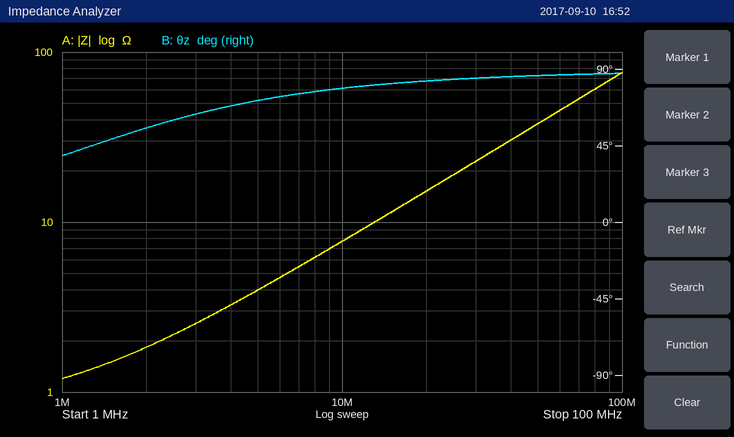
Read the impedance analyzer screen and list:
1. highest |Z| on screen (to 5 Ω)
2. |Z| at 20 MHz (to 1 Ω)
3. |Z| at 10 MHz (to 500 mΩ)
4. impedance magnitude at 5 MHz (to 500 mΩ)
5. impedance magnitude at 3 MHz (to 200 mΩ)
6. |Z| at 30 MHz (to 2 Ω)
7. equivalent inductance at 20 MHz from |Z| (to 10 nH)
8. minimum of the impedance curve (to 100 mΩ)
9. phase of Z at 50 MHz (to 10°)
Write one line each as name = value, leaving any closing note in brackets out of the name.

highest |Z| on screen = 75 Ω
|Z| at 20 MHz = 15 Ω
|Z| at 10 MHz = 7.5 Ω
impedance magnitude at 5 MHz = 4.0 Ω
impedance magnitude at 3 MHz = 2.6 Ω
|Z| at 30 MHz = 22 Ω
equivalent inductance at 20 MHz from |Z| = 120 nH
minimum of the impedance curve = 1.2 Ω
phase of Z at 50 MHz = 90°
